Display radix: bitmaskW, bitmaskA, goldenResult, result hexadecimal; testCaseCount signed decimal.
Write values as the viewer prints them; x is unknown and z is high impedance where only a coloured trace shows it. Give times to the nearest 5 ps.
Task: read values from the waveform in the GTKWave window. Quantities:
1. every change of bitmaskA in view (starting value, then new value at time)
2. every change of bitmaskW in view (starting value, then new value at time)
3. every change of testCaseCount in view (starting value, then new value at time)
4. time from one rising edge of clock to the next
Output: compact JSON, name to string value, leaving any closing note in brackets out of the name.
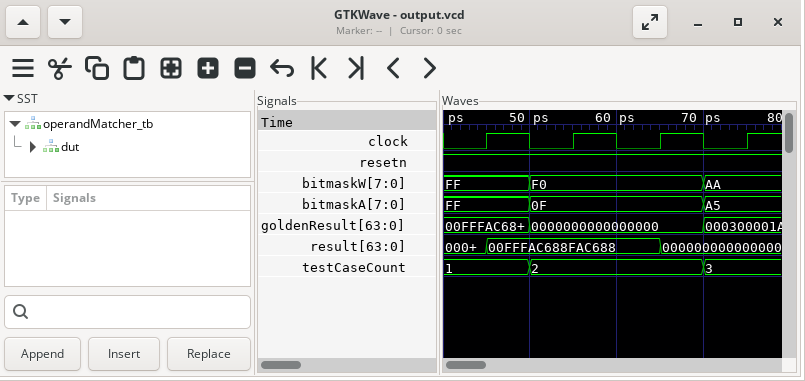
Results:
{"every change of bitmaskA in view": "FF, 0F at 50 ps, A5 at 70 ps", "every change of bitmaskW in view": "FF, F0 at 50 ps, AA at 70 ps", "every change of testCaseCount in view": "1, 2 at 50 ps, 3 at 70 ps", "time from one rising edge of clock to the next": "10 ps"}
